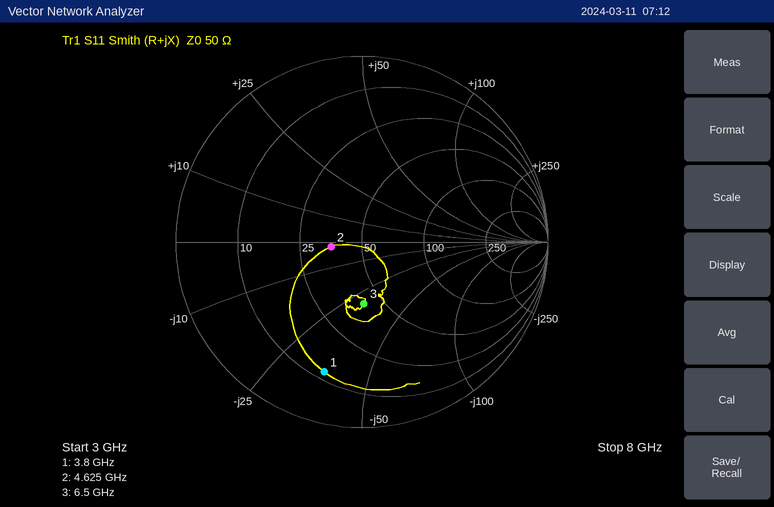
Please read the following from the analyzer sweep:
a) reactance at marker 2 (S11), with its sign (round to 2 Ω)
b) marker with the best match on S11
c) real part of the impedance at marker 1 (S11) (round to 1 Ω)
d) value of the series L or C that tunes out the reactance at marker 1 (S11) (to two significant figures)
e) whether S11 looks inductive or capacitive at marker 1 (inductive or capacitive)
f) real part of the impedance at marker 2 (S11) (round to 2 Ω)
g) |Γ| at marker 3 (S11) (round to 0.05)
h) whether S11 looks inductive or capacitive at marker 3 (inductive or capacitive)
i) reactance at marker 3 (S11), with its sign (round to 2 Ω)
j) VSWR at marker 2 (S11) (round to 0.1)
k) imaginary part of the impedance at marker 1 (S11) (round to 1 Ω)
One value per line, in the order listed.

-2 Ω
marker 2
12 Ω
1.5 nH
capacitive
36 Ω
0.35
capacitive
-30 Ω
1.4
-36 Ω
